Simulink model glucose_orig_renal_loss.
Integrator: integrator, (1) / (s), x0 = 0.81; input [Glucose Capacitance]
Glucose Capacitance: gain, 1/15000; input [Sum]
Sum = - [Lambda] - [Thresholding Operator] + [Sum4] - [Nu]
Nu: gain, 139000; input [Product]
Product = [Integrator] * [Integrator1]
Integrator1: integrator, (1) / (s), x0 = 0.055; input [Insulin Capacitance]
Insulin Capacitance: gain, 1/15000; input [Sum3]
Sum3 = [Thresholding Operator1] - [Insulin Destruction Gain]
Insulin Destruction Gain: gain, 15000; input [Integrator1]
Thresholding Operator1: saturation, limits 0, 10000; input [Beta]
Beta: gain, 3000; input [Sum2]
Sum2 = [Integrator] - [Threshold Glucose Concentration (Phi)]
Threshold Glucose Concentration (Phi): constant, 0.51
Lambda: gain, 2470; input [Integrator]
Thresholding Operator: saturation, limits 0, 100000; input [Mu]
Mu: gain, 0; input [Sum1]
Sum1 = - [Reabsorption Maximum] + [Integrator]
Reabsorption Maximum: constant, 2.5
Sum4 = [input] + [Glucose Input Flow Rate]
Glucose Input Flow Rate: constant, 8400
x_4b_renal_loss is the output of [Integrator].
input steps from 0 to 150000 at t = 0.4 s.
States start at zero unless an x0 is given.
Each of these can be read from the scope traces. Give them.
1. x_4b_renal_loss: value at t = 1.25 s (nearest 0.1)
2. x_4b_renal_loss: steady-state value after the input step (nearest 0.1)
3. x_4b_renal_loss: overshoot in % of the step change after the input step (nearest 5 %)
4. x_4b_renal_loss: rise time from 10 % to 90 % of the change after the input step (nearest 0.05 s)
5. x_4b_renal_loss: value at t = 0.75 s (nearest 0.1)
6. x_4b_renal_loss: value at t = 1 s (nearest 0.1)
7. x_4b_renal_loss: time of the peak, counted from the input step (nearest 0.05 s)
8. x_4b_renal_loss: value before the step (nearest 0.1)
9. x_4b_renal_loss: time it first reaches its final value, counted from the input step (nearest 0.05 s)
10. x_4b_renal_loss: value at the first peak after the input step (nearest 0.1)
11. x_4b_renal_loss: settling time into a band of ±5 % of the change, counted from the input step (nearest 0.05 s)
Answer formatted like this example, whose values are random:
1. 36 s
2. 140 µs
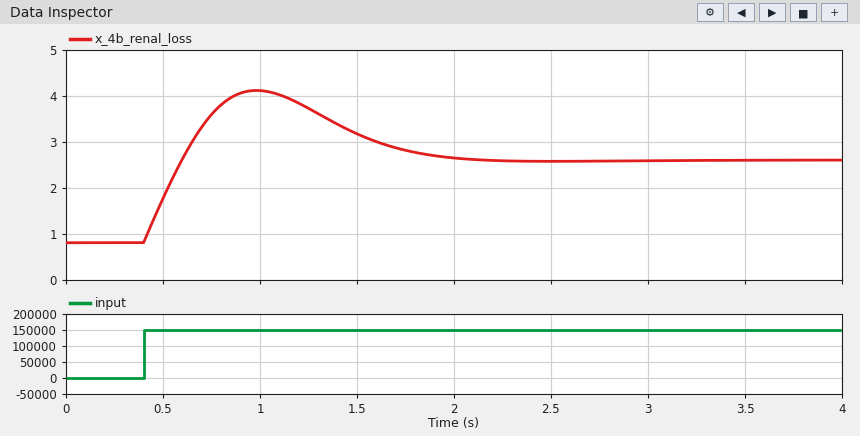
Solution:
1. 3.7
2. 2.6
3. 85 %
4. 0.15 s
5. 3.6
6. 4.1
7. 0.60 s
8. 0.8
9. 0.20 s
10. 4.1
11. 1.50 s
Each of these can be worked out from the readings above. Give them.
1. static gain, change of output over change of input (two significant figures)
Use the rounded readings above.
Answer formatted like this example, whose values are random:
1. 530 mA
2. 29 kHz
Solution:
1. 0.000012
